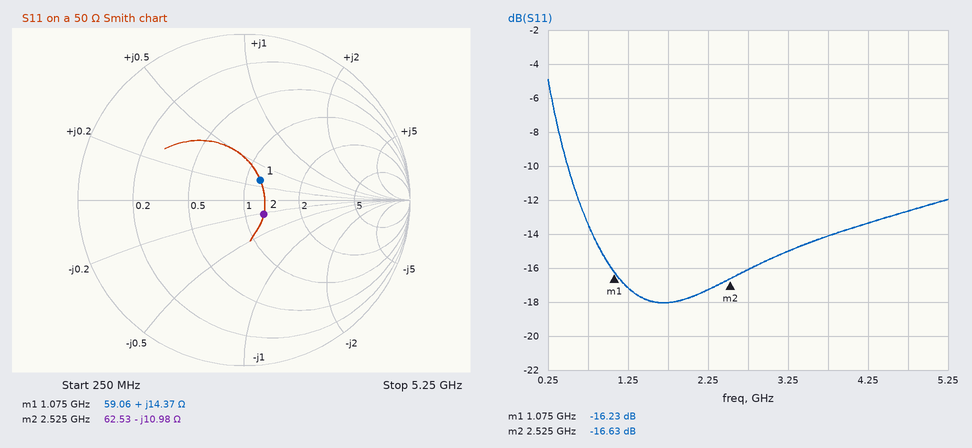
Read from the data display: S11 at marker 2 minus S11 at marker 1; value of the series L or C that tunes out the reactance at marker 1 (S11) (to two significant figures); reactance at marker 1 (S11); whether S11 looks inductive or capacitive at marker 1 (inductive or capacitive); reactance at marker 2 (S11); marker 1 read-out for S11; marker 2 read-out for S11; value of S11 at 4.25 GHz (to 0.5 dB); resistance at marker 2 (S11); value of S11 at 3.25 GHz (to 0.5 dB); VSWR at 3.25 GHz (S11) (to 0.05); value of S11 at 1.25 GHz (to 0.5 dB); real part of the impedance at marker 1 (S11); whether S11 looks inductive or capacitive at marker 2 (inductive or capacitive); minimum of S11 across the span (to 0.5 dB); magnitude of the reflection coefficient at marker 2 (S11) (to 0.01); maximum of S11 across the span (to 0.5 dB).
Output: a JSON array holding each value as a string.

["-0.40 dB", "10 pF", "+14.37 Ω", "inductive", "-10.98 Ω", "-16.23 dB", "-16.63 dB", "-13.5 dB", "62.53 Ω", "-15.0 dB", "1.45", "-17.0 dB", "59.06 Ω", "capacitive", "-18.0 dB", "0.15", "-5.0 dB"]
